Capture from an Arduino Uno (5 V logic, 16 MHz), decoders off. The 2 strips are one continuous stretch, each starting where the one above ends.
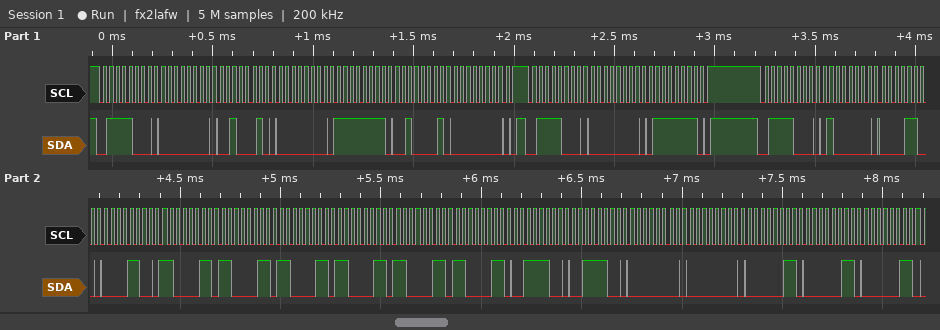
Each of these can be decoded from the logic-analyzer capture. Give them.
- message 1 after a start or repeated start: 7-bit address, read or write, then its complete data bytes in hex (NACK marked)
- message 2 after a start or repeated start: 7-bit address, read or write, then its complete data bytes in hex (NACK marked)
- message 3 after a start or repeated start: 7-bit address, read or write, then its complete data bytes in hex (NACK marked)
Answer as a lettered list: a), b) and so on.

a) 0x3C write: 00 22 00 FF 21 00
b) 0x3C write: 00 7F
c) 0x3C write: 40 0C 0C C3 C3 C3 C3 C3 C3 3C 3C 00 00 03 03 03
